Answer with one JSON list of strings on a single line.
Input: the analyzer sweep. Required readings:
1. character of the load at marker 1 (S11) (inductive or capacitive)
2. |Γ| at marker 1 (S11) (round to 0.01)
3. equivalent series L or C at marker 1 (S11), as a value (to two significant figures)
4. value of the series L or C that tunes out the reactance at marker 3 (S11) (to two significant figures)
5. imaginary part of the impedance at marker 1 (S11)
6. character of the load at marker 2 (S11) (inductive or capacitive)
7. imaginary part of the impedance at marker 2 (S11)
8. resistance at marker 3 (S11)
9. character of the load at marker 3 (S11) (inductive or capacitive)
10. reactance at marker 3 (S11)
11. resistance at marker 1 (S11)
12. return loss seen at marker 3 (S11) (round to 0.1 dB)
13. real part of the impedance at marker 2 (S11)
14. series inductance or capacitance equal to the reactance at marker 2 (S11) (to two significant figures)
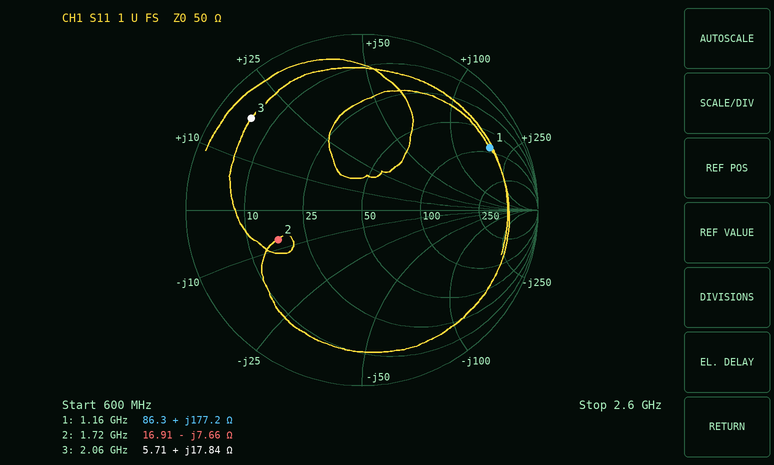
["inductive", "0.81", "24 nH", "4.3 pF", "+177.2 Ω", "capacitive", "-7.66 Ω", "5.71 Ω", "inductive", "+17.84 Ω", "86.3 Ω", "1.8 dB", "16.91 Ω", "12 pF"]
